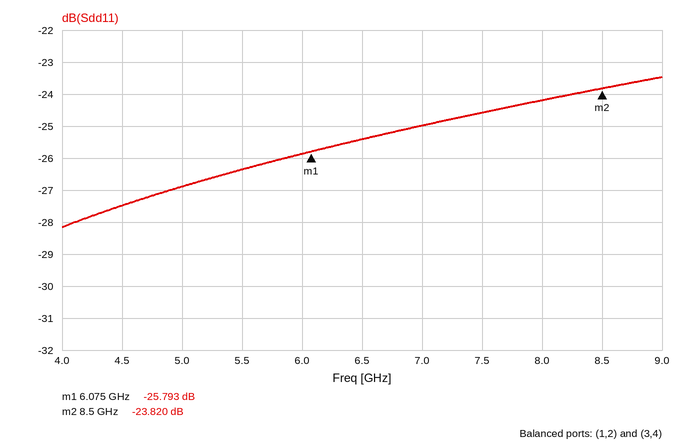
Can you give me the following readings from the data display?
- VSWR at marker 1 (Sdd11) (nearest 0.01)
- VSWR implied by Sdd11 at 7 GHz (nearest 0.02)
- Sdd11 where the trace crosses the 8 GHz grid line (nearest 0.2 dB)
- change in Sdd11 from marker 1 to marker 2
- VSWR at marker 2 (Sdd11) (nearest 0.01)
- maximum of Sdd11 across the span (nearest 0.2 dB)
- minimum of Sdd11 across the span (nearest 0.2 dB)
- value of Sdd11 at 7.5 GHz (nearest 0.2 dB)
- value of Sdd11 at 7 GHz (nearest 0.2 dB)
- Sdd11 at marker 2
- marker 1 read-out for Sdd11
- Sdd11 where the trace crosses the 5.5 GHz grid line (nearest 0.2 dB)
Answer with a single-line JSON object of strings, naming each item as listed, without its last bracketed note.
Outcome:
{"VSWR at marker 1 (Sdd11)": "1.11", "VSWR implied by Sdd11 at 7 GHz": "1.12", "Sdd11 where the trace crosses the 8 GHz grid line": "-24.2 dB", "change in Sdd11 from marker 1 to marker 2": "1.973 dB", "VSWR at marker 2 (Sdd11)": "1.14", "maximum of Sdd11 across the span": "-23.4 dB", "minimum of Sdd11 across the span": "-28.2 dB", "value of Sdd11 at 7.5 GHz": "-24.6 dB", "value of Sdd11 at 7 GHz": "-25.0 dB", "Sdd11 at marker 2": "-23.820 dB", "marker 1 read-out for Sdd11": "-25.793 dB", "Sdd11 where the trace crosses the 5.5 GHz grid line": "-26.4 dB"}
